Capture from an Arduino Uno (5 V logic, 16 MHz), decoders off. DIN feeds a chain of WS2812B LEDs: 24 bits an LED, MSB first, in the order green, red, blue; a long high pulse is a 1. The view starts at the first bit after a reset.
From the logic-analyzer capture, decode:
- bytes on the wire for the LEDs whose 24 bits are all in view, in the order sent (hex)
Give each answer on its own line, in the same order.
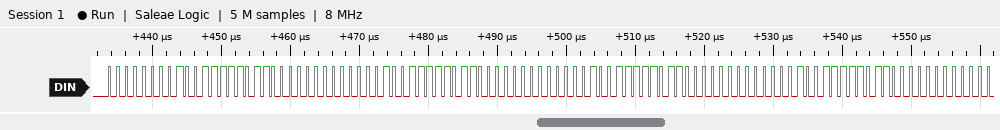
00 9F 60 00 9F 60 00 9F 60 00 9F 60
